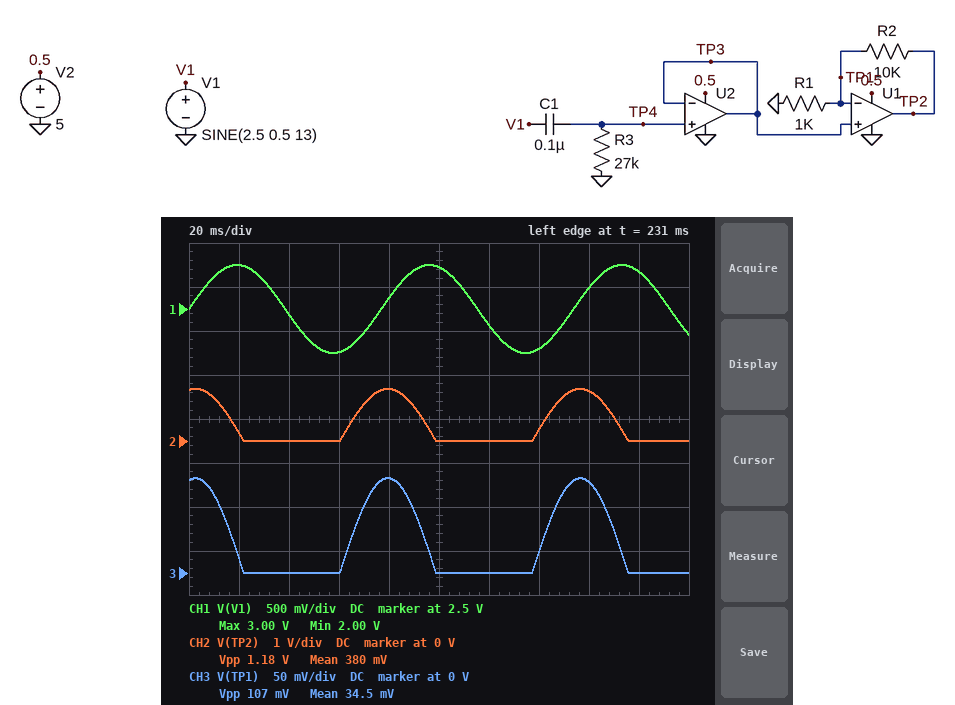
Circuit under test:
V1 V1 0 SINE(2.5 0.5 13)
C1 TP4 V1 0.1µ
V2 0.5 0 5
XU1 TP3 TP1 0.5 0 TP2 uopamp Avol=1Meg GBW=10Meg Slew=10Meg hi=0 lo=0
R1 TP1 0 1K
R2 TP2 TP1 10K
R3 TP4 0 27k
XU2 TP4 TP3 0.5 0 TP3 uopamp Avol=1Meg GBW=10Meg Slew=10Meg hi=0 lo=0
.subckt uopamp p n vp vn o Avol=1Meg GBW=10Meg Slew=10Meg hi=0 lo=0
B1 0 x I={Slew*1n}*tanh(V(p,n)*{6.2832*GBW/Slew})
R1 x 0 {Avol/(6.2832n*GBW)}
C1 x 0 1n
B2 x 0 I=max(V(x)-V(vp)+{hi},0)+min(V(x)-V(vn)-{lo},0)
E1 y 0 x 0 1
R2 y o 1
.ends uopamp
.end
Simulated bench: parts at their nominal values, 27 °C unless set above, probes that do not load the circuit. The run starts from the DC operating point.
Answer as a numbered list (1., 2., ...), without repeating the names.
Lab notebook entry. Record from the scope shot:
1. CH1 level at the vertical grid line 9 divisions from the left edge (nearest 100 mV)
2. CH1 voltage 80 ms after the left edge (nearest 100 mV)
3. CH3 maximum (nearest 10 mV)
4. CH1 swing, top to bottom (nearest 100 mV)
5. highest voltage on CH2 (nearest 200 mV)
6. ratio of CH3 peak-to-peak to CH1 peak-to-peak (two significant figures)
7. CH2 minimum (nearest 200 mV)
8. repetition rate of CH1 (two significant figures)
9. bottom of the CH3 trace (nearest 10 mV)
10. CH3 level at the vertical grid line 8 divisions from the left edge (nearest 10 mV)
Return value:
1. 2.9 V
2. 2.6 V
3. 110 mV
4. 1.0 V
5. 1.2 V
6. 0.11
7. 0 V
8. 13 Hz
9. 0 V
10. 100 mV
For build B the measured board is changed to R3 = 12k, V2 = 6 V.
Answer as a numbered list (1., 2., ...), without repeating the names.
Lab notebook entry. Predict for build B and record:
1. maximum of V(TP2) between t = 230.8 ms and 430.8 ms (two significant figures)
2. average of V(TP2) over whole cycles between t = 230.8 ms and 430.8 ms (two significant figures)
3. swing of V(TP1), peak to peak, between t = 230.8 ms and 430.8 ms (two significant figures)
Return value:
1. 540 mV
2. 170 mV
3. 49 mV
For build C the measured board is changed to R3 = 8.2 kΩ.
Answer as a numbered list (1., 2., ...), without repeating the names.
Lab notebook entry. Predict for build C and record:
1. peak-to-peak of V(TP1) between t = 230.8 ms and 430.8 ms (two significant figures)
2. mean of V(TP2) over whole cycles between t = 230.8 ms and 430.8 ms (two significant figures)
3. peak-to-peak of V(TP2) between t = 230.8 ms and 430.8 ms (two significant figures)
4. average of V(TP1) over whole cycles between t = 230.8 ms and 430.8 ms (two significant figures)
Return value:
1. 33 mV
2. 120 mV
3. 370 mV
4. 11 mV
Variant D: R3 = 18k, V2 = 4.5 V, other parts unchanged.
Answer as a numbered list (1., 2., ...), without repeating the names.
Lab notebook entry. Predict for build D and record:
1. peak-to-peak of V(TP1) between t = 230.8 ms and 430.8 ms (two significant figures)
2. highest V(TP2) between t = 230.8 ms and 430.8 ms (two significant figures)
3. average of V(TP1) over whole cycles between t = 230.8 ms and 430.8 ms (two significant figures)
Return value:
1. 73 mV
2. 800 mV
3. 23 mV
